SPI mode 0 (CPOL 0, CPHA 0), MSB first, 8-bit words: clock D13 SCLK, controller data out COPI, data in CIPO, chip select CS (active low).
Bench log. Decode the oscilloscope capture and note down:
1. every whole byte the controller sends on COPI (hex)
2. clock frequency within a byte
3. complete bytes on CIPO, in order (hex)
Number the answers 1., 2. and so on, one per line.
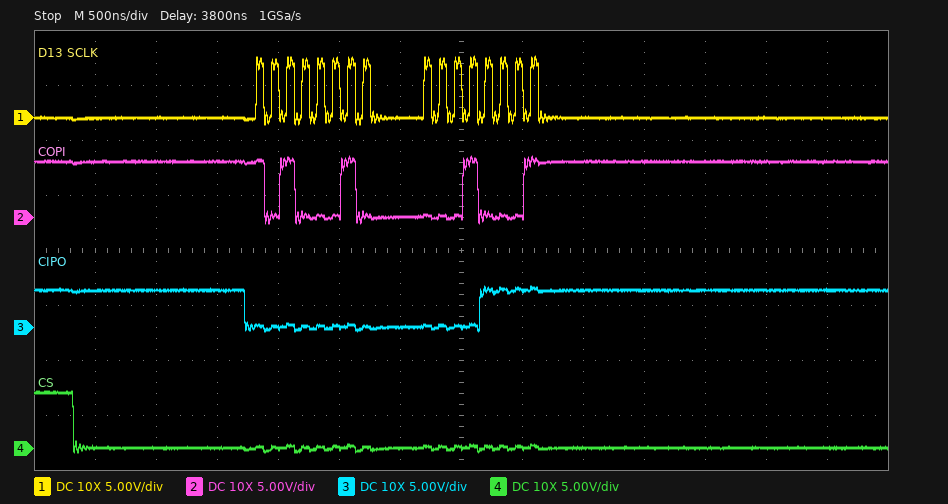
1. A2 11
2. 8 MHz
3. 00 0F
